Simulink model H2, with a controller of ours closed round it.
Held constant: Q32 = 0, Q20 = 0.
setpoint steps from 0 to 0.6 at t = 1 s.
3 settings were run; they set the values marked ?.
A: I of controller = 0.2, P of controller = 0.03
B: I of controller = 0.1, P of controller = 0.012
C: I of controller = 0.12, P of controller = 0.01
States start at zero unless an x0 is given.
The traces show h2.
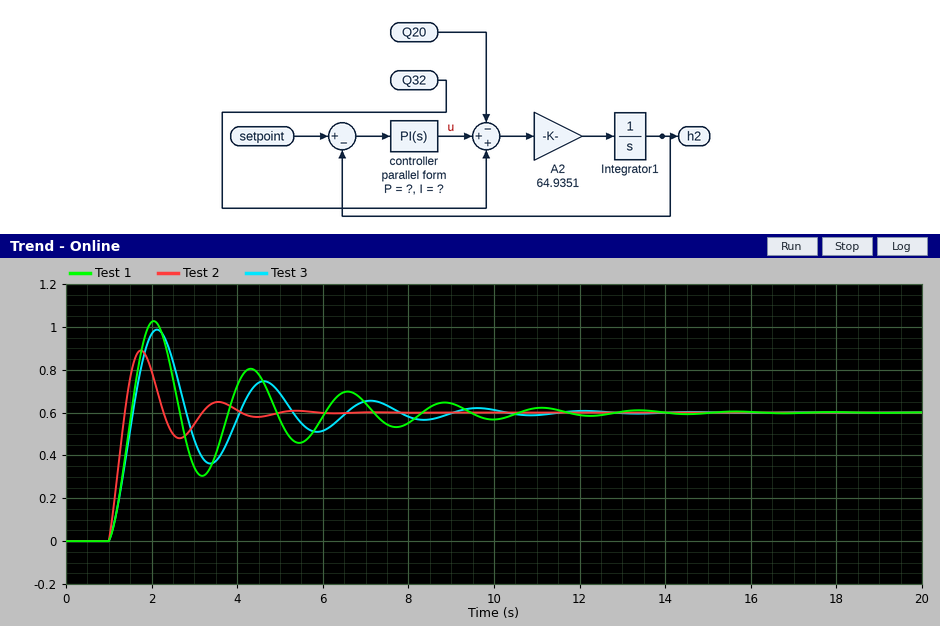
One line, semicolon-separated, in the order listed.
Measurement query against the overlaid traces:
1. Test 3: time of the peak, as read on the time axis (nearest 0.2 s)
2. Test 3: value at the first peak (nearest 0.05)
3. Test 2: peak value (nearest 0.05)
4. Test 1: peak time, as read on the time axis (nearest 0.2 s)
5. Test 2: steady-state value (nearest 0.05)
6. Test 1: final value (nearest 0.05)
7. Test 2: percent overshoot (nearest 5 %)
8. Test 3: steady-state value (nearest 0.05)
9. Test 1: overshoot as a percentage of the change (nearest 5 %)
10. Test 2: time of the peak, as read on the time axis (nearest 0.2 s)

2.2 s; 1.00; 0.90; 2.0 s; 0.60; 0.60; 50 %; 0.60; 70 %; 1.8 s
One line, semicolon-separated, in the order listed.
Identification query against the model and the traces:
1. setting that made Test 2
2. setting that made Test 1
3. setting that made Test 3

A; C; B
